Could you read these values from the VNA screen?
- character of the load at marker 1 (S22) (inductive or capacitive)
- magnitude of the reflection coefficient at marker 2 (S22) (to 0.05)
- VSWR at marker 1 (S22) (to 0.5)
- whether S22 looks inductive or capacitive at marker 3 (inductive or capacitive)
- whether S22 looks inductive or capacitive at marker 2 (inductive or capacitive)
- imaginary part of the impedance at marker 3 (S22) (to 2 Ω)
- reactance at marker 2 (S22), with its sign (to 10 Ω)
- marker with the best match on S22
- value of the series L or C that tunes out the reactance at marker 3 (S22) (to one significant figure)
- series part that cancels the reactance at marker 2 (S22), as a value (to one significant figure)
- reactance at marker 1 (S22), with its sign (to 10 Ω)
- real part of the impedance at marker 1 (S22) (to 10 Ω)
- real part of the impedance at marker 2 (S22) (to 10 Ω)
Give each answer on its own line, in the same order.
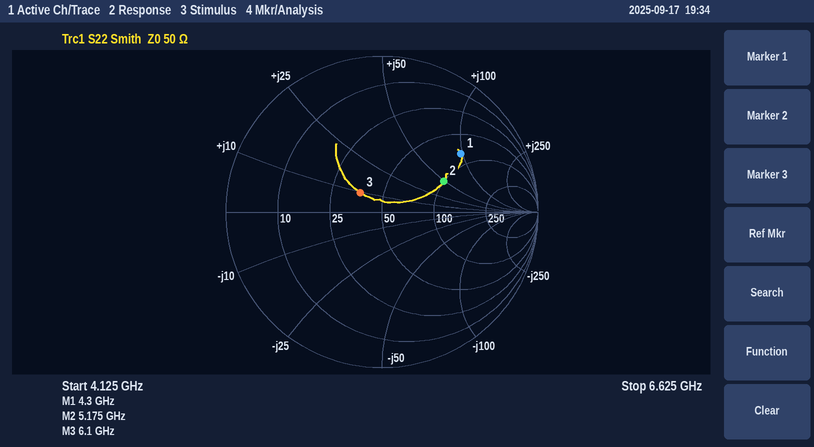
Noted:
inductive
0.45
4.5
inductive
inductive
+10 Ω
+50 Ω
marker 3
3 pF
600 fF
+100 Ω
80 Ω
100 Ω
